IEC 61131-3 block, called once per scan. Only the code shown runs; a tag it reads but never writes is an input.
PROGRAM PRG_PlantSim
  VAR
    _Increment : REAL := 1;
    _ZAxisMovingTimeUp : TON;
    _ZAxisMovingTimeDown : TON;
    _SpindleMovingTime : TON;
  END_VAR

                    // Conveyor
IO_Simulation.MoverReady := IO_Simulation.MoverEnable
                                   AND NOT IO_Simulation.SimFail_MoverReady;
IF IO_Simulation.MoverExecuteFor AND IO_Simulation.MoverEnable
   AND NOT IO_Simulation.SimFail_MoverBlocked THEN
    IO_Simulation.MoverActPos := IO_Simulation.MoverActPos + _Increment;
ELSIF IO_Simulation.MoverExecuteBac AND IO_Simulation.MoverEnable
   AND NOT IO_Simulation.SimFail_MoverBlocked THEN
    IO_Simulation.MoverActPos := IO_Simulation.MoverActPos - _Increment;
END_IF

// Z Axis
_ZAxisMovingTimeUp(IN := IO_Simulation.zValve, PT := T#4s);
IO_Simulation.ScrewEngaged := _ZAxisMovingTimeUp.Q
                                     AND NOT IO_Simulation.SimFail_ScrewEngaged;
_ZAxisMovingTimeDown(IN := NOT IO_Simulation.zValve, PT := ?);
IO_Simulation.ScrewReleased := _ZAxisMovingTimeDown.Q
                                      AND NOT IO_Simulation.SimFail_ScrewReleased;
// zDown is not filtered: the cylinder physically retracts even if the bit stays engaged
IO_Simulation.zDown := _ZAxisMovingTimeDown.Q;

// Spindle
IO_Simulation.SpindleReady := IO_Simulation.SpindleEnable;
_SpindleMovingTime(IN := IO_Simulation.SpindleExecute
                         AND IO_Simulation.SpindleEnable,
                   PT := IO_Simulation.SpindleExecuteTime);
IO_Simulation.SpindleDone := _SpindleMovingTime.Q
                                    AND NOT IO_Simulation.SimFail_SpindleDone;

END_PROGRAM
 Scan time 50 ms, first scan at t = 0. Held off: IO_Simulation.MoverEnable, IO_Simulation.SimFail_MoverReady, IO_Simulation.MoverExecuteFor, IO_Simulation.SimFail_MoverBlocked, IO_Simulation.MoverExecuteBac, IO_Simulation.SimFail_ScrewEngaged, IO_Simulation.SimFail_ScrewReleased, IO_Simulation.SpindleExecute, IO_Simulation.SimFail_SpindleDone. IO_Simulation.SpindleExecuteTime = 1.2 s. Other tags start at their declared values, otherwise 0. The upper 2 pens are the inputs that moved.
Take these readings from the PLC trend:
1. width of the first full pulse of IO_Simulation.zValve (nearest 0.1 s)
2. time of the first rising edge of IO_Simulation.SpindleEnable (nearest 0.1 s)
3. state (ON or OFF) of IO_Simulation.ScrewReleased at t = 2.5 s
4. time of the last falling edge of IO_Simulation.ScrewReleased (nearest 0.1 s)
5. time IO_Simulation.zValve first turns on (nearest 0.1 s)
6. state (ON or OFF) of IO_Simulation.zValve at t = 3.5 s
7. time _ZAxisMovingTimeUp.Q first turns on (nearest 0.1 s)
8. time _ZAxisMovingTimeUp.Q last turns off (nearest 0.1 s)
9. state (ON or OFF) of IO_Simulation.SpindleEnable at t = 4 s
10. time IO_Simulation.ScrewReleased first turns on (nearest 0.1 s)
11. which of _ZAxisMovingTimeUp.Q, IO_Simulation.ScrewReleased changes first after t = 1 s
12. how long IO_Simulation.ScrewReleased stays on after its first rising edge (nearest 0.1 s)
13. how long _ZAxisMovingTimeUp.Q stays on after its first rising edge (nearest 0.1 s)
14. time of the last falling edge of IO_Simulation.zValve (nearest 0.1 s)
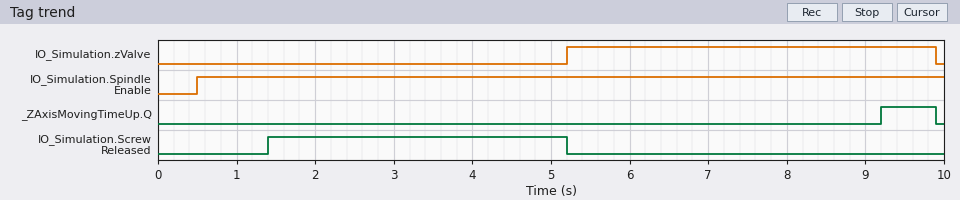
4.7 s
0.5 s
ON
5.2 s
5.2 s
OFF
9.2 s
9.9 s
ON
1.4 s
IO_Simulation.ScrewReleased
3.8 s
0.7 s
9.9 s
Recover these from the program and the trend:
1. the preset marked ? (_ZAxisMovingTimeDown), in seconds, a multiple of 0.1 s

1.4 s
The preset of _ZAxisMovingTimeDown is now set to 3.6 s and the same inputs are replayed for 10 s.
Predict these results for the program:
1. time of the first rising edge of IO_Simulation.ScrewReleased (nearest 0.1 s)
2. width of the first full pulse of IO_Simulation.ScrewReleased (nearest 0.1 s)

3.6 s
1.6 s
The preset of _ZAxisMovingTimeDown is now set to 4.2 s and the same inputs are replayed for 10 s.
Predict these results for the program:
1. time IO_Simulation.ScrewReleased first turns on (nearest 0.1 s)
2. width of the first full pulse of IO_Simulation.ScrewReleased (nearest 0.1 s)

4.2 s
1.0 s
